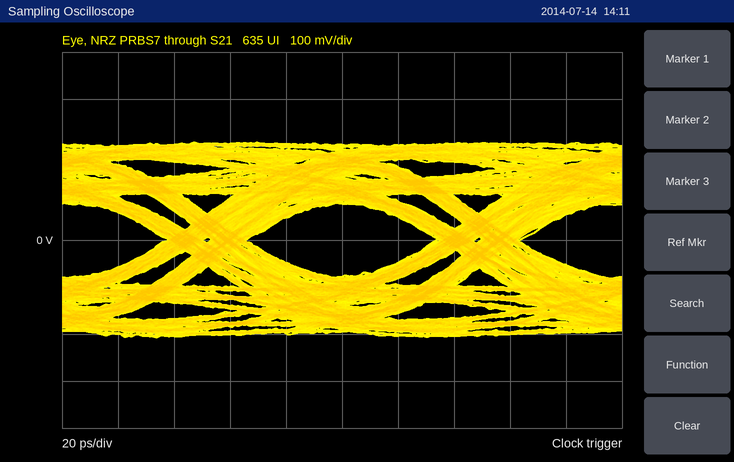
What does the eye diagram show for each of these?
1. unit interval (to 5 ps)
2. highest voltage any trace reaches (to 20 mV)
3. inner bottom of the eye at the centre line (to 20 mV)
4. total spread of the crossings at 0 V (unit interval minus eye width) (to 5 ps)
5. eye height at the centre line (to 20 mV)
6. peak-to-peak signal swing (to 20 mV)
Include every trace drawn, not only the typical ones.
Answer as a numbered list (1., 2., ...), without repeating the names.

1. 95 ps
2. 200 mV
3. -80 mV
4. 30 ps
5. 160 mV
6. 420 mV
